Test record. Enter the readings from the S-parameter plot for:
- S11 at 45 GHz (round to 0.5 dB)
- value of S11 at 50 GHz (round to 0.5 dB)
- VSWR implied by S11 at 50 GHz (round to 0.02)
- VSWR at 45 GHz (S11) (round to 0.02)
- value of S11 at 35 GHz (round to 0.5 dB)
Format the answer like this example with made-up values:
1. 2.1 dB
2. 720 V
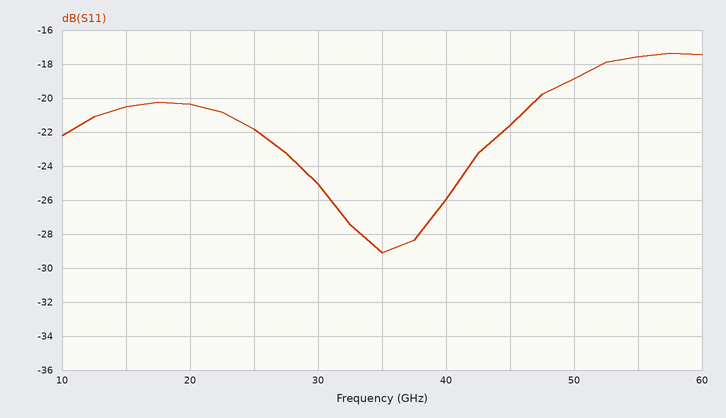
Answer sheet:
1. -21.5 dB
2. -19.0 dB
3. 1.26
4. 1.18
5. -29.0 dB
